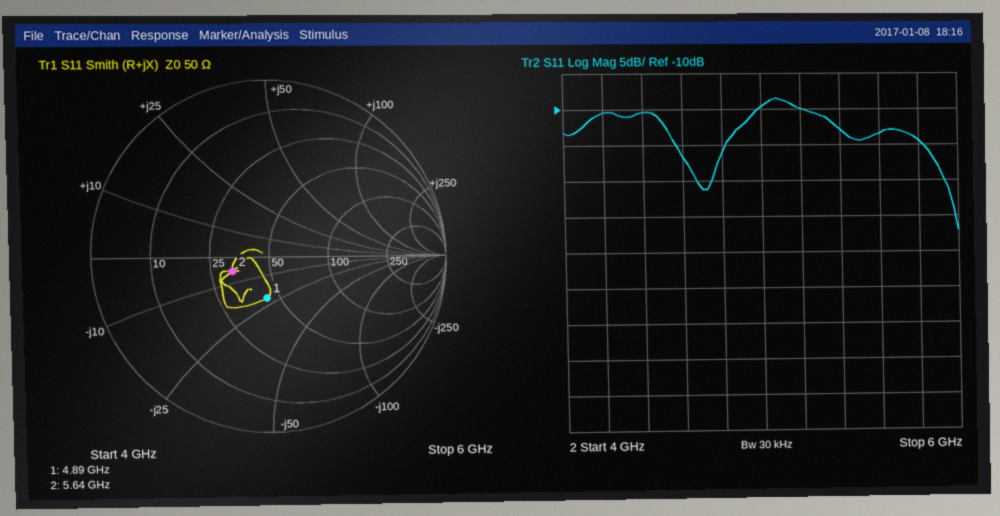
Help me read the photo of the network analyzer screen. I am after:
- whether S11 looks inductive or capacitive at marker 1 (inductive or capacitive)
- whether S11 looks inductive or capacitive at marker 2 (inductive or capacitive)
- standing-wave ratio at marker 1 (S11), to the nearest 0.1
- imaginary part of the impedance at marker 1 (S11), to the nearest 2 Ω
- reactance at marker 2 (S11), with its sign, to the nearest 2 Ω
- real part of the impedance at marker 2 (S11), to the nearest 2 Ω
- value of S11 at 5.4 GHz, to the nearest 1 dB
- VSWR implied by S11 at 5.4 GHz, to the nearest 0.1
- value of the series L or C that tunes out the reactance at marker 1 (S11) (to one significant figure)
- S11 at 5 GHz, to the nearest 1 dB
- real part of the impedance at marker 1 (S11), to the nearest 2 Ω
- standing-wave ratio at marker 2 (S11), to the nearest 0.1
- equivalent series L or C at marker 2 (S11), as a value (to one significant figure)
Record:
capacitive
capacitive
1.6
-22 Ω
-6 Ω
32 Ω
-13 dB
1.6
700 pH
-10 dB
44 Ω
1.6
5 pF
